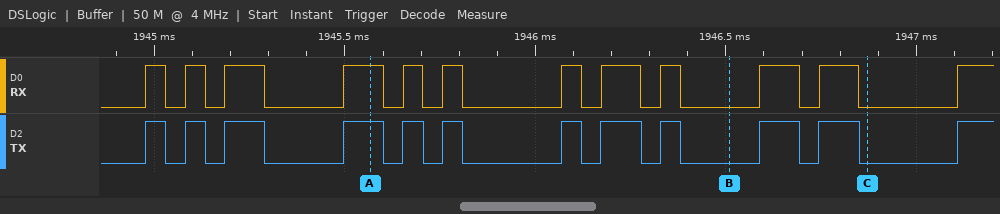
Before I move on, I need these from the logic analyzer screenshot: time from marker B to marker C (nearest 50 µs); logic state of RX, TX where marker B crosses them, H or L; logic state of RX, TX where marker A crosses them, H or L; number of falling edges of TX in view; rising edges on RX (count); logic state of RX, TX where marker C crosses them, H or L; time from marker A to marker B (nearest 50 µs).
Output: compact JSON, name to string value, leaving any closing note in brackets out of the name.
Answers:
{"time from marker B to marker C": "350 µs", "logic state of RX, TX where marker B crosses them, H or L": "RX=L, TX=L", "logic state of RX, TX where marker A crosses them, H or L": "RX=H, TX=H", "number of falling edges of TX in view": "11", "rising edges on RX": "12", "logic state of RX, TX where marker C crosses them, H or L": "RX=L, TX=L", "time from marker A to marker B": "950 µs"}
